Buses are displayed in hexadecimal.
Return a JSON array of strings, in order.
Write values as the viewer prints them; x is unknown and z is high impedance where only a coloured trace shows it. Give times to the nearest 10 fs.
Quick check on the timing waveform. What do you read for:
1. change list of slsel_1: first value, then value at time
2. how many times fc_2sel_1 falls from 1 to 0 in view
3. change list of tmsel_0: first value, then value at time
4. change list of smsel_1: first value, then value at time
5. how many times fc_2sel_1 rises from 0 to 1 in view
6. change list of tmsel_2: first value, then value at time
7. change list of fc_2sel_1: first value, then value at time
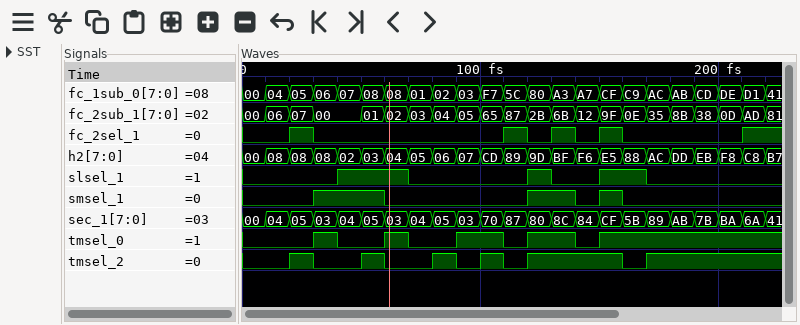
["0, 1 at 40 fs, 0 at 70 fs, 1 at 120 fs, 0 at 130 fs, 1 at 150 fs, 0 at 170 fs", "4", "0, 1 at 30 fs, 0 at 40 fs, 1 at 60 fs, 0 at 70 fs, 1 at 90 fs, 0 at 110 fs, 1 at 120 fs, 0 at 140 fs, 1 at 150 fs", "0, 1 at 30 fs, 0 at 60 fs, 1 at 120 fs, 0 at 140 fs, 1 at 150 fs, 0 at 160 fs", "5", "0, 1 at 20 fs, 0 at 30 fs, 1 at 50 fs, 0 at 60 fs, 1 at 80 fs, 0 at 90 fs, 1 at 100 fs, 0 at 110 fs, 1 at 120 fs, 0 at 160 fs, 1 at 170 fs", "0, 1 at 20 fs, 0 at 30 fs, 1 at 110 fs, 0 at 120 fs, 1 at 130 fs, 0 at 140 fs, 1 at 150 fs, 0 at 160 fs, 1 at 210 fs"]
